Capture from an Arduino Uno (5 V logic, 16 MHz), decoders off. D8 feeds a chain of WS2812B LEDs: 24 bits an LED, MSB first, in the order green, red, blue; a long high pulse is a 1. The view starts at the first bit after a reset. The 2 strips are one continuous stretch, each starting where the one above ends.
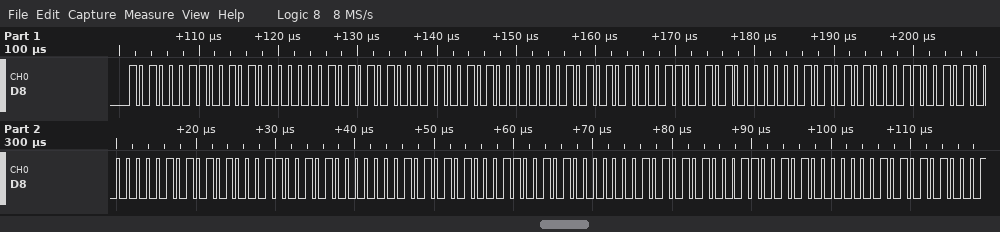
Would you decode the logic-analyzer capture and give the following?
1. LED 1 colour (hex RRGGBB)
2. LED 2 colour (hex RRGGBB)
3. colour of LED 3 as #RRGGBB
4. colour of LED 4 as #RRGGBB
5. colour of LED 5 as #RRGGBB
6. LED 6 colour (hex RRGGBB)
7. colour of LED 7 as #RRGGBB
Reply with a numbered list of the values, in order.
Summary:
1. #28A30A
2. #28A30A
3. #28A30A
4. #28A30A
5. #28A30A
6. #28A30A
7. #28A30A
